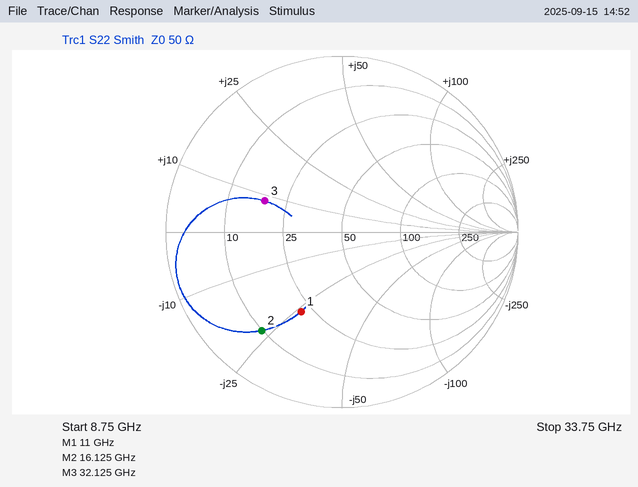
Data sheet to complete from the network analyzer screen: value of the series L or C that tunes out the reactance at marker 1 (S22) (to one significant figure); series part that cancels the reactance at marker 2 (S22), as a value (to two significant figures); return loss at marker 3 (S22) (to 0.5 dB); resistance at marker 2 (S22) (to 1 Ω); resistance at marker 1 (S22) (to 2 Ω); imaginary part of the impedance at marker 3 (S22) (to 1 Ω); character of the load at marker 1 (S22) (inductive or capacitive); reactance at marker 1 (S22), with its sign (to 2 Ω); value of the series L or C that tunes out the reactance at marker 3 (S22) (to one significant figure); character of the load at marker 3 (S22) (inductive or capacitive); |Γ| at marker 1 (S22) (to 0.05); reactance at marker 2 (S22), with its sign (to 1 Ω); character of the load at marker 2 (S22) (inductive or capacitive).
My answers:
400 pH
230 pH
6.5 dB
10 Ω
22 Ω
+8 Ω
capacitive
-26 Ω
600 fF
inductive
0.50
-23 Ω
capacitive
